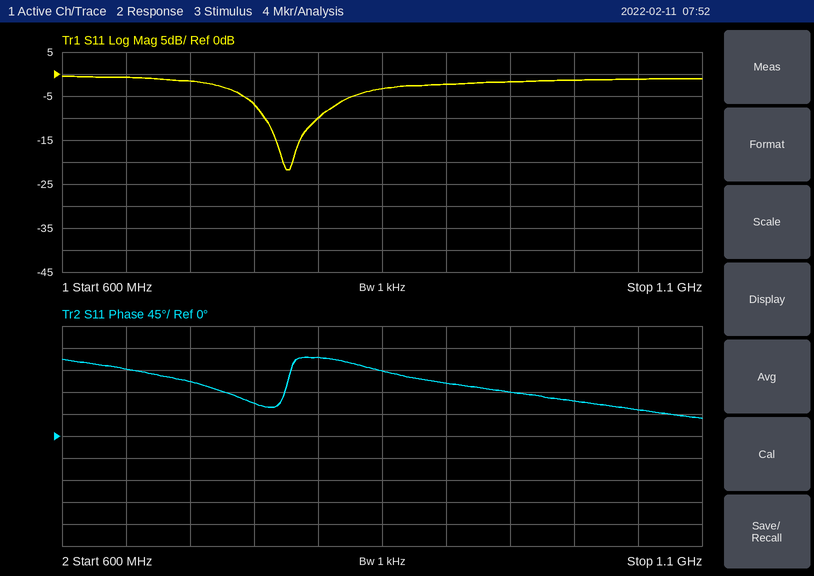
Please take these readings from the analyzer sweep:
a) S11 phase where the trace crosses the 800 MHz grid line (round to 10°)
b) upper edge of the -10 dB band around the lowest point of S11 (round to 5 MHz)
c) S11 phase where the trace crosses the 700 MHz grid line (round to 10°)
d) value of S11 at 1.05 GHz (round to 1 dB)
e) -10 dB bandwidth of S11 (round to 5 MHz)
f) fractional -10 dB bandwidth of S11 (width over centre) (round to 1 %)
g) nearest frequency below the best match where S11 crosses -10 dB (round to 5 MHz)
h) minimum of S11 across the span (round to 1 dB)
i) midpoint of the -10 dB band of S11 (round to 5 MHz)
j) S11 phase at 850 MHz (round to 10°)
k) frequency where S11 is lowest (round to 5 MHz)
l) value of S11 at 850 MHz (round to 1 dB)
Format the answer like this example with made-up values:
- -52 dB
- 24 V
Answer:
- 160°
- 800 MHz
- 110°
- -1 dB
- 40 MHz
- 5 %
- 760 MHz
- -22 dB
- 780 MHz
- 130°
- 775 MHz
- -3 dB
